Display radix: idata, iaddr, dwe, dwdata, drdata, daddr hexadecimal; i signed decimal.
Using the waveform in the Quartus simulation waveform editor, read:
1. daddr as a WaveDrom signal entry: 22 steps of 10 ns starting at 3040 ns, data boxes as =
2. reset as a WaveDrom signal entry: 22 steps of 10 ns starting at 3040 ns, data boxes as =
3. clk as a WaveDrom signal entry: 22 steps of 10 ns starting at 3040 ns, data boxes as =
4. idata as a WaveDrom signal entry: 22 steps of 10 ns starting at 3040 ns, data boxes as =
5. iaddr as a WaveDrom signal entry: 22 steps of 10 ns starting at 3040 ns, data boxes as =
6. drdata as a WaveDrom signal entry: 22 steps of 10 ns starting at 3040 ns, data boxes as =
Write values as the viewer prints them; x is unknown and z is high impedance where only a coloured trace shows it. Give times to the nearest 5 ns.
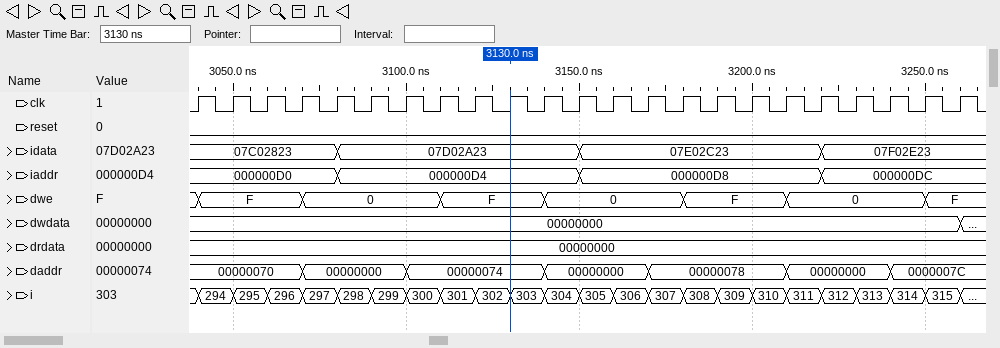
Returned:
{name: 'daddr', wave: '=..=..=...=..=...=..=.', data: '00000070 00000000 00000074 00000000 00000078 00000000 0000007C'}
{name: 'reset', wave: '0.....................'}
{name: 'clk', wave: 'p.....................'}
{name: 'idata', wave: '=...=......=......=...', data: '07C02823 07D02A23 07E02C23 07F02E23'}
{name: 'iaddr', wave: '=...=......=......=...', data: '000000D0 000000D4 000000D8 000000DC'}
{name: 'drdata', wave: '=.....................', data: '00000000'}
